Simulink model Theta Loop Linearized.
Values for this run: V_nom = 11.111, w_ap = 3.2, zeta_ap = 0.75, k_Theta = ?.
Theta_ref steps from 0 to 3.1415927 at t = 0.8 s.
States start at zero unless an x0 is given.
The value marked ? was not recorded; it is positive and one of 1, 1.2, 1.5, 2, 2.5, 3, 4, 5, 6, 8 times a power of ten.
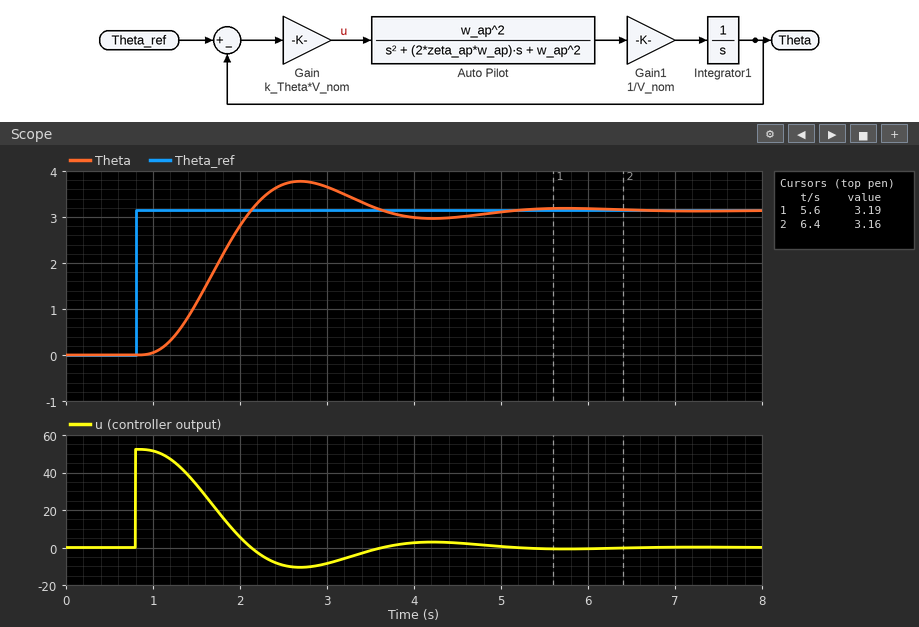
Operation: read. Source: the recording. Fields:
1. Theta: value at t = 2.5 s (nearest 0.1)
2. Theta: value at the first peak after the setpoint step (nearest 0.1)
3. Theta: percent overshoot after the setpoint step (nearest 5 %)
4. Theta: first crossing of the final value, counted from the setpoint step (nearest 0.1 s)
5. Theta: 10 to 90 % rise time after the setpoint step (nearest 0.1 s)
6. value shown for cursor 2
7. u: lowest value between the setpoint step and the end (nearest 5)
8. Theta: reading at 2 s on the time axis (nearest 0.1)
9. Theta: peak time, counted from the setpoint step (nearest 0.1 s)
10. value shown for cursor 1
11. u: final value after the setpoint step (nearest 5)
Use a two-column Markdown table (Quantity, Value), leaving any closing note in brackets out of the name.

| Quantity | Value |
|---|---|
| Theta: value at t = 2.5 s | 3.7 |
| Theta: value at the first peak after the setpoint step | 3.8 |
| Theta: percent overshoot after the setpoint step | 20 % |
| Theta: first crossing of the final value, counted from the setpoint step | 1.3 s |
| Theta: 10 to 90 % rise time after the setpoint step | 0.8 s |
| value shown for cursor 2 | 3.16 |
| u: lowest value between the setpoint step and the end | -10 |
| Theta: reading at 2 s on the time axis | 2.8 |
| Theta: peak time, counted from the setpoint step | 1.9 s |
| value shown for cursor 1 | 3.19 |
| u: final value after the setpoint step | 0 |
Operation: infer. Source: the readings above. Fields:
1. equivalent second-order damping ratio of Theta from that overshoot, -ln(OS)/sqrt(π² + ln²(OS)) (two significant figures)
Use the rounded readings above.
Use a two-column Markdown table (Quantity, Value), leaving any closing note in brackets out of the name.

| Quantity | Value |
|---|---|
| equivalent second-order damping ratio of Theta from that overshoot, -ln(OS)/sqrt(π² + ln²(OS)) | 0.46 |
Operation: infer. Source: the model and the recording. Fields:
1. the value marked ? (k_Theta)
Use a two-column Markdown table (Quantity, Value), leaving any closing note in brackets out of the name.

| Quantity | Value |
|---|---|
| the value marked ? | 1.5 |
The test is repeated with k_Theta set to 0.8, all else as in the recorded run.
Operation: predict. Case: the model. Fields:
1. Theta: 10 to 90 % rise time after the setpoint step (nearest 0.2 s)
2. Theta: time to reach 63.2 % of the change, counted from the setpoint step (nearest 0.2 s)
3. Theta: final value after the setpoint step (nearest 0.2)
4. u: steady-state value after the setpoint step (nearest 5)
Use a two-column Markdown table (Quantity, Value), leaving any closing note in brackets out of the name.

| Quantity | Value |
|---|---|
| Theta: 10 to 90 % rise time after the setpoint step | 1.6 s |
| Theta: time to reach 63.2 % of the change, counted from the setpoint step | 1.4 s |
| Theta: final value after the setpoint step | 3.2 |
| u: steady-state value after the setpoint step | 0 |
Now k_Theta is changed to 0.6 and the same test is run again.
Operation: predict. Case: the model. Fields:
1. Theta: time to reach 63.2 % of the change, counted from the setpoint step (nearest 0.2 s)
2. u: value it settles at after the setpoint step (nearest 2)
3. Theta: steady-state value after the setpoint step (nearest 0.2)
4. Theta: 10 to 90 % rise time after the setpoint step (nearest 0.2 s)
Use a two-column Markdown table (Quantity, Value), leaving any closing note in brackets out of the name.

| Quantity | Value |
|---|---|
| Theta: time to reach 63.2 % of the change, counted from the setpoint step | 1.8 s |
| u: value it settles at after the setpoint step | 0 |
| Theta: steady-state value after the setpoint step | 3.2 |
| Theta: 10 to 90 % rise time after the setpoint step | 2.4 s |
